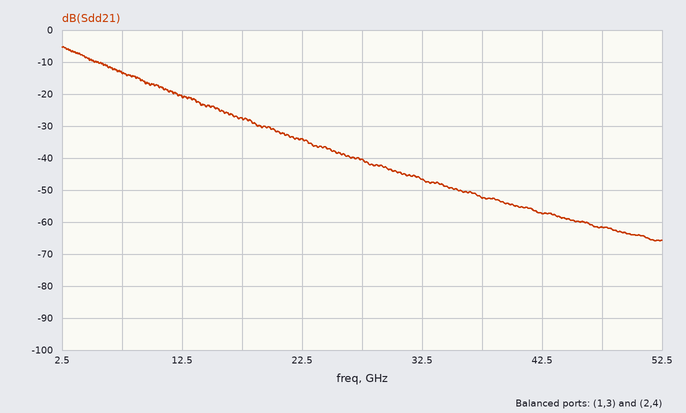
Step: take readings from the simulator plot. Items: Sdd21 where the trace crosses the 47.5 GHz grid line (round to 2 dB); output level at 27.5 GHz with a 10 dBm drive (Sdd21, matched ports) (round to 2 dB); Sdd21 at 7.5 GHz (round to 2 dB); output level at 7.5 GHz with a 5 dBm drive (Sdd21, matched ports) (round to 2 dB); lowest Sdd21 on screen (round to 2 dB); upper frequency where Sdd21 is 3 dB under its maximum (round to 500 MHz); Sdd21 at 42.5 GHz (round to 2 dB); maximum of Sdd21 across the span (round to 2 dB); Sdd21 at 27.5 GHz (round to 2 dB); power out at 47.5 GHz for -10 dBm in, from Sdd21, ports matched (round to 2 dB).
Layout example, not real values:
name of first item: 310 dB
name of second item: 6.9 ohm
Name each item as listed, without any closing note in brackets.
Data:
Sdd21 where the trace crosses the 47.5 GHz grid line: -62 dB
output level at 27.5 GHz with a 10 dBm drive (Sdd21, matched ports): -30 dBm
Sdd21 at 7.5 GHz: -14 dB
output level at 7.5 GHz with a 5 dBm drive (Sdd21, matched ports): -8 dBm
lowest Sdd21 on screen: -66 dB
upper frequency where Sdd21 is 3 dB under its maximum: 4.5 GHz
Sdd21 at 42.5 GHz: -58 dB
maximum of Sdd21 across the span: -6 dB
Sdd21 at 27.5 GHz: -40 dB
power out at 47.5 GHz for -10 dBm in, from Sdd21, ports matched: -72 dBm
